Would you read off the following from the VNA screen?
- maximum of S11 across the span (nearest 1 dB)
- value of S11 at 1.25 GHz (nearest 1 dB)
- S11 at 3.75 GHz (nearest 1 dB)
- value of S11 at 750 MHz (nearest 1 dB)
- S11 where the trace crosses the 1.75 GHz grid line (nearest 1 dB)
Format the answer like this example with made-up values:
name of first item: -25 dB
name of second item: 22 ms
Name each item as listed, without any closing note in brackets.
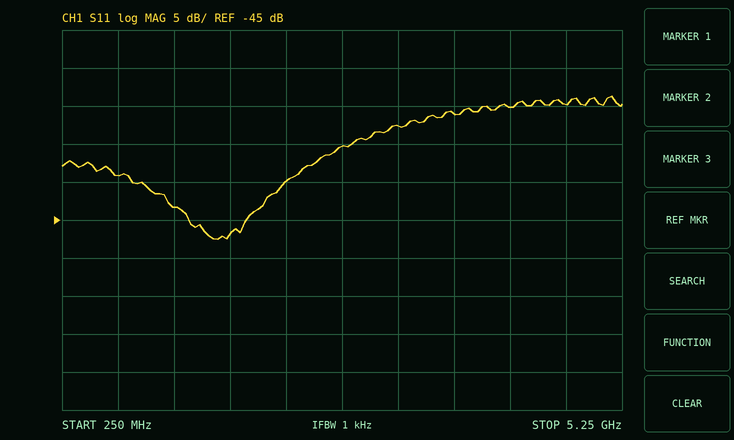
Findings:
maximum of S11 across the span: -29 dB
value of S11 at 1.25 GHz: -43 dB
S11 at 3.75 GHz: -31 dB
value of S11 at 750 MHz: -39 dB
S11 where the trace crosses the 1.75 GHz grid line: -47 dB
